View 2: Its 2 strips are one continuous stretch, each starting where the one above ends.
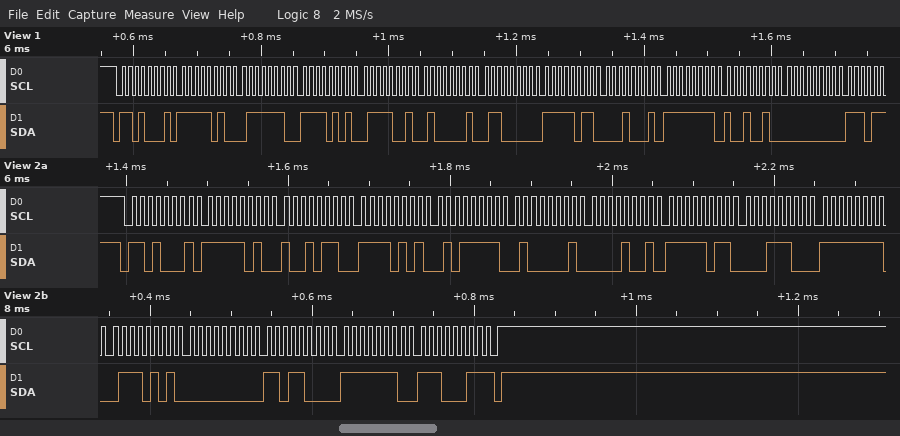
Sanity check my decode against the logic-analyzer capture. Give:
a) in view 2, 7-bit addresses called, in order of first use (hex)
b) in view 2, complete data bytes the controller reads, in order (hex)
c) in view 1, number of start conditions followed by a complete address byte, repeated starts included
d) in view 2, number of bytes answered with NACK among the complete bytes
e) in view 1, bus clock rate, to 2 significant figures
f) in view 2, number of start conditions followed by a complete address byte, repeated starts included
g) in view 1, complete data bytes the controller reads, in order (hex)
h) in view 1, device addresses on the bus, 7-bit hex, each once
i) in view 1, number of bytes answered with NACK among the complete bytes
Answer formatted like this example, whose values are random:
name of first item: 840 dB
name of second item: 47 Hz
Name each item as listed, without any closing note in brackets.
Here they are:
in view 2, 7-bit addresses called, in order of first use: 0x68
in view 2, complete data bytes the controller reads, in order: FA 96 F5 5F 41 09 FB 1C FF 75 00 D8 FE E3
in view 1, number of start conditions followed by a complete address byte, repeated starts included: 1
in view 2, number of bytes answered with NACK among the complete bytes: 1
in view 1, bus clock rate, to 2 significant figures: 100 kHz
in view 2, number of start conditions followed by a complete address byte, repeated starts included: 1
in view 1, complete data bytes the controller reads, in order: FA 7E F5 79 41 60 FB 11 FF 92 00
in view 1, device addresses on the bus, 7-bit hex, each once: 0x68
in view 1, number of bytes answered with NACK among the complete bytes: 0
